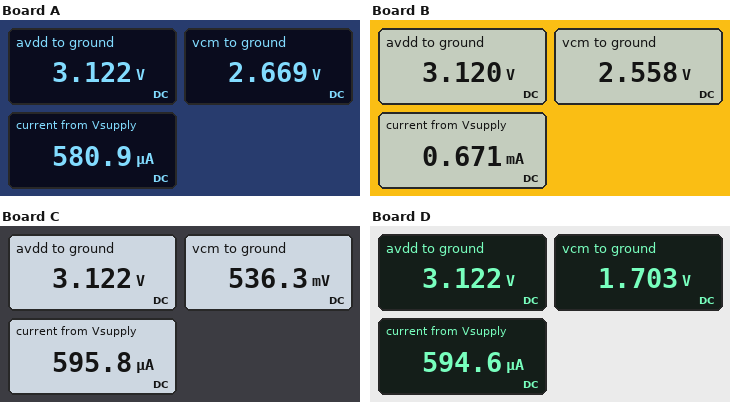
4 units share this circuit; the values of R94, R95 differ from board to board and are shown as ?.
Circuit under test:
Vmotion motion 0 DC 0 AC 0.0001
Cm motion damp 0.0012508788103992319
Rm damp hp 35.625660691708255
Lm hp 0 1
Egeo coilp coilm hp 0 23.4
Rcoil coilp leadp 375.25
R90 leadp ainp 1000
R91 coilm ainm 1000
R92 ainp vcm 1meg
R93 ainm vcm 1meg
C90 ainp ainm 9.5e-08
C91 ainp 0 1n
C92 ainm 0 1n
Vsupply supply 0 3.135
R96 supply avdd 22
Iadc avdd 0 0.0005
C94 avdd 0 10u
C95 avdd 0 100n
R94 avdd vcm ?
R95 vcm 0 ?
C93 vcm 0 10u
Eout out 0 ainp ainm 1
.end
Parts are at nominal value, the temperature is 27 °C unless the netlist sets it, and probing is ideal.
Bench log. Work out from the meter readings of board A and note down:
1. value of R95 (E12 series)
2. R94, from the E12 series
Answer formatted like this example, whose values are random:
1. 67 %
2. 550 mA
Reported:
1. 33 kΩ
2. 5.6 kΩ
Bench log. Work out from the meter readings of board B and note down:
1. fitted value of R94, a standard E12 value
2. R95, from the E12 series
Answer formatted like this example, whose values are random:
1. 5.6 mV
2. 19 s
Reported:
1. 3.3 kΩ
2. 15 kΩ
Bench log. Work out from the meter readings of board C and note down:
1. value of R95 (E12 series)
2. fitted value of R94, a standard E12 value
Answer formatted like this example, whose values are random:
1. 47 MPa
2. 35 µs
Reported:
1. 5.6 kΩ
2. 27 kΩ
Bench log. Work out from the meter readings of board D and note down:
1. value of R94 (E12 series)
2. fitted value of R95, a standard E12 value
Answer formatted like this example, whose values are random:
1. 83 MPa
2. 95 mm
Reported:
1. 15 kΩ
2. 18 kΩ
